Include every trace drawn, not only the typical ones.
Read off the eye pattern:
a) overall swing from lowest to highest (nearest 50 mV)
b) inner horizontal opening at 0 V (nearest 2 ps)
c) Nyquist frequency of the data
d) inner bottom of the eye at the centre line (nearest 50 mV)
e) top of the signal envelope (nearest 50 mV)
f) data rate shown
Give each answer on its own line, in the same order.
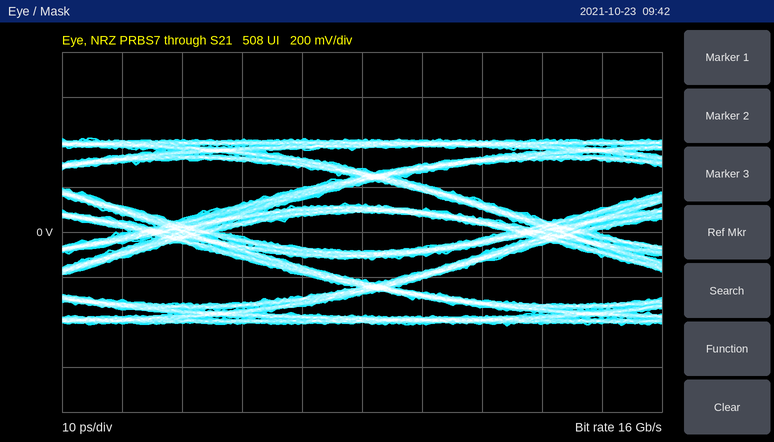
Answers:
850 mV
48 ps
8 GHz
-100 mV
400 mV
16 Gb/s
